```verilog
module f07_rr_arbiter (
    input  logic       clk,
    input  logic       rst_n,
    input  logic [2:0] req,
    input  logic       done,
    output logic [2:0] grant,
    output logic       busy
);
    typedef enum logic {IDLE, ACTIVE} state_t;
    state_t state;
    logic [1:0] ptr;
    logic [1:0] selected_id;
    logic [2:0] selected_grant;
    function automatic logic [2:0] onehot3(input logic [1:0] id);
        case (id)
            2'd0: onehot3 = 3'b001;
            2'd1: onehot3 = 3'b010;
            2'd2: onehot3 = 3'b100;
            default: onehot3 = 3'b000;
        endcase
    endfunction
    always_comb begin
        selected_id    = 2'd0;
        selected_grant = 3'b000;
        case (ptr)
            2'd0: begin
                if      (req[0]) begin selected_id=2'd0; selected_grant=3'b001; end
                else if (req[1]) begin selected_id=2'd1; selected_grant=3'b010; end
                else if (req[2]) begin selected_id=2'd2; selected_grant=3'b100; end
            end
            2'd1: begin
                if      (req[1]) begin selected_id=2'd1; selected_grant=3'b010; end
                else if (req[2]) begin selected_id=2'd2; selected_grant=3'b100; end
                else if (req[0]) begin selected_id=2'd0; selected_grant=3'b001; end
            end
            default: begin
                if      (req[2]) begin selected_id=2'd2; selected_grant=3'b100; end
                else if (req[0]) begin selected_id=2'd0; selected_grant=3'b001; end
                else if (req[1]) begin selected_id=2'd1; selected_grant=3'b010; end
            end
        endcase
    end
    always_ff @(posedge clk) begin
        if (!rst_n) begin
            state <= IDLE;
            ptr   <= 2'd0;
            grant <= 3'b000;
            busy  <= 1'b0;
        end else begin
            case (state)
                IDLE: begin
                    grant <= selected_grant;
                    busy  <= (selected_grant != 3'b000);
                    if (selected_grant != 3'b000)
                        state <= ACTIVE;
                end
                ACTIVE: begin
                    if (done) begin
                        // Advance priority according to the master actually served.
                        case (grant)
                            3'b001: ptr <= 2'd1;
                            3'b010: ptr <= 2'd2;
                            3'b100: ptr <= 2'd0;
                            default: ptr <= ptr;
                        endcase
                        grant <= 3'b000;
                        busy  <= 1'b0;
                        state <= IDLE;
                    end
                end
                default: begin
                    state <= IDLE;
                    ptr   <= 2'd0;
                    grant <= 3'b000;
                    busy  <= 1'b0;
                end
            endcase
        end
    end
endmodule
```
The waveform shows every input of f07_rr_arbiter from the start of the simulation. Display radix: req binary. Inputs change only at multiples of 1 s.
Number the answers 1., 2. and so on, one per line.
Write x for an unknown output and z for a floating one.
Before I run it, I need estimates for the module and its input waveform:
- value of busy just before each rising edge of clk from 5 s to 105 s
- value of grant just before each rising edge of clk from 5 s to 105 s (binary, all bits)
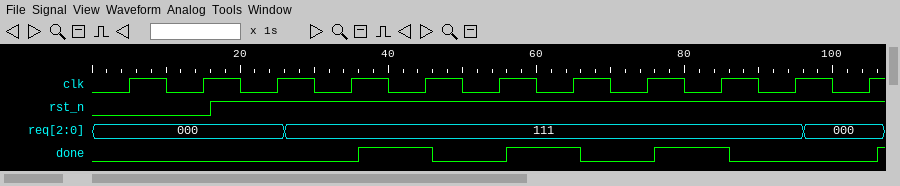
1. x 0 0 0 1 0 1 0 1 0 1
2. x, 000, 000, 000, 001, 000, 010, 000, 100, 000, 001
